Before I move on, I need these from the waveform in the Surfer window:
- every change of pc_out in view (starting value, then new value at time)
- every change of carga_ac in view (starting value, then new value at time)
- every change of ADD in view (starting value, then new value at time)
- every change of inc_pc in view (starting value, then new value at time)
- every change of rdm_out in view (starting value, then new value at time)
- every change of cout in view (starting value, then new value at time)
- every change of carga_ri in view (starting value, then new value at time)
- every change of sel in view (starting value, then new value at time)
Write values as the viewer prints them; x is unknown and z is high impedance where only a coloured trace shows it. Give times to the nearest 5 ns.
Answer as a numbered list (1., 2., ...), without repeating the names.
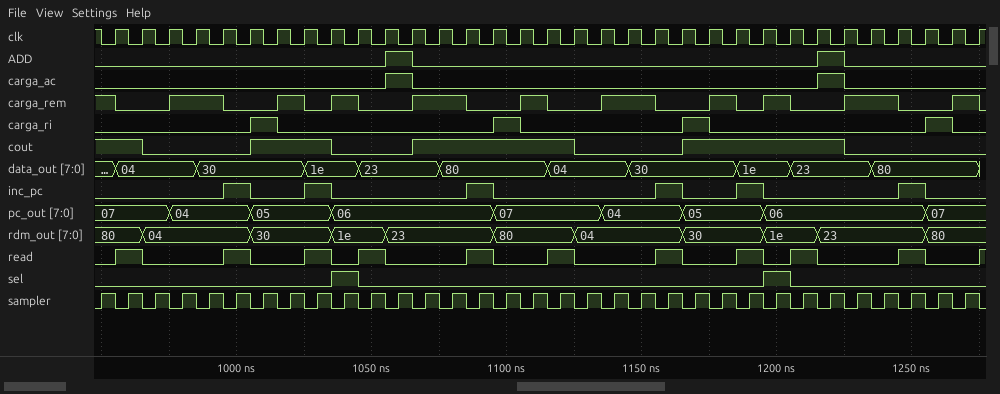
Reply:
1. 07, 04 at 975 ns, 05 at 1005 ns, 06 at 1035 ns, 07 at 1095 ns, 04 at 1135 ns, 05 at 1165 ns, 06 at 1195 ns, 07 at 1255 ns
2. 0, 1 at 1055 ns, 0 at 1065 ns, 1 at 1215 ns, 0 at 1225 ns
3. 0, 1 at 1055 ns, 0 at 1065 ns, 1 at 1215 ns, 0 at 1225 ns
4. 0, 1 at 995 ns, 0 at 1005 ns, 1 at 1025 ns, 0 at 1035 ns, 1 at 1085 ns, 0 at 1095 ns, 1 at 1155 ns, 0 at 1165 ns, 1 at 1185 ns, 0 at 1195 ns, 1 at 1245 ns, 0 at 1255 ns
5. 80, 04 at 965 ns, 30 at 1005 ns, 1e at 1035 ns, 23 at 1055 ns, 80 at 1095 ns, 04 at 1125 ns, 30 at 1165 ns, 1e at 1195 ns, 23 at 1215 ns, 80 at 1255 ns
6. 1, 0 at 965 ns, 1 at 1005 ns, 0 at 1035 ns, 1 at 1065 ns, 0 at 1125 ns, 1 at 1165 ns, 0 at 1225 ns
7. 0, 1 at 1005 ns, 0 at 1015 ns, 1 at 1095 ns, 0 at 1105 ns, 1 at 1165 ns, 0 at 1175 ns, 1 at 1255 ns, 0 at 1265 ns
8. 0, 1 at 1035 ns, 0 at 1045 ns, 1 at 1195 ns, 0 at 1205 ns
